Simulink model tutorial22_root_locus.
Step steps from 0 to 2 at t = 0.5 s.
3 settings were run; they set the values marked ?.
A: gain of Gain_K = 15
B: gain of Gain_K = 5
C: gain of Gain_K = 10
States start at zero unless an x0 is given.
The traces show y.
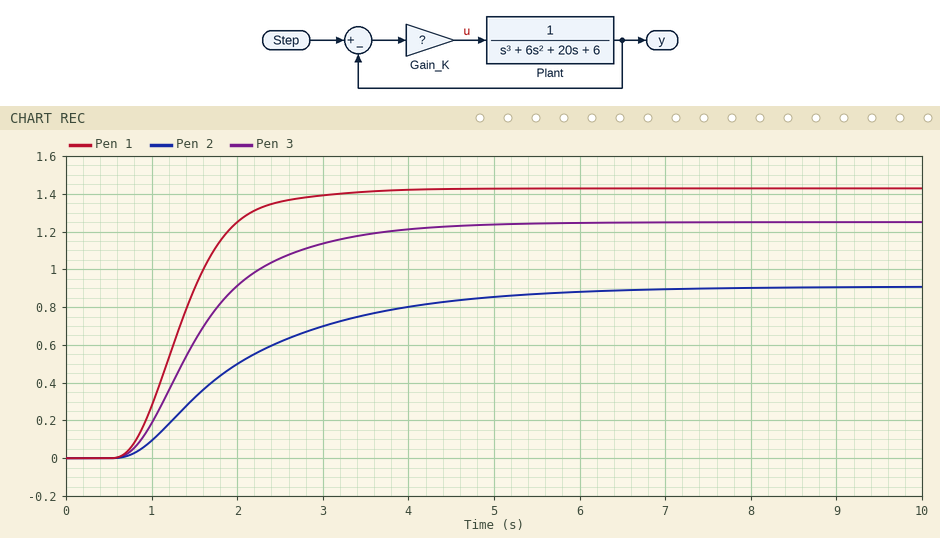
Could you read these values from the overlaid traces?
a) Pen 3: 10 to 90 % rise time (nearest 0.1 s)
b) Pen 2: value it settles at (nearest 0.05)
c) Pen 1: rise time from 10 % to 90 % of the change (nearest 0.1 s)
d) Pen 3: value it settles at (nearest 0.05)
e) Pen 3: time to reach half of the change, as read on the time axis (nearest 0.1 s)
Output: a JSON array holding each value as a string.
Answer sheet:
["2.0 s", "0.90", "1.2 s", "1.25", "1.5 s"]
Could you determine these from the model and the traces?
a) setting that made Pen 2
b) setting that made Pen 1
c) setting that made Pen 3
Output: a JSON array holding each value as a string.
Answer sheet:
["B", "A", "C"]
